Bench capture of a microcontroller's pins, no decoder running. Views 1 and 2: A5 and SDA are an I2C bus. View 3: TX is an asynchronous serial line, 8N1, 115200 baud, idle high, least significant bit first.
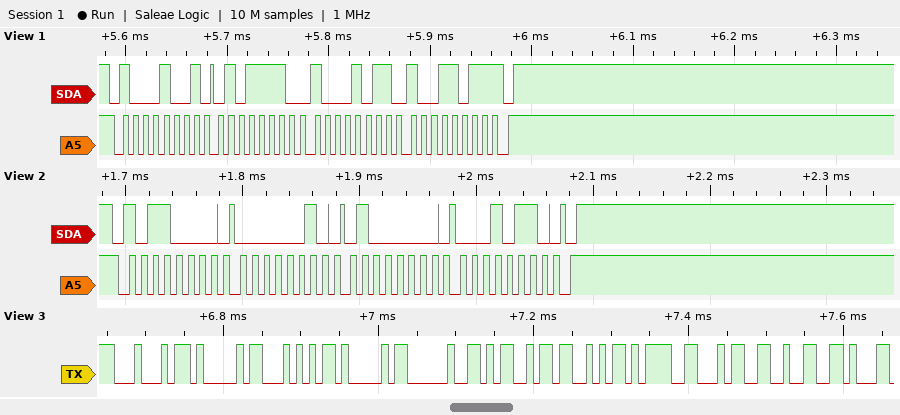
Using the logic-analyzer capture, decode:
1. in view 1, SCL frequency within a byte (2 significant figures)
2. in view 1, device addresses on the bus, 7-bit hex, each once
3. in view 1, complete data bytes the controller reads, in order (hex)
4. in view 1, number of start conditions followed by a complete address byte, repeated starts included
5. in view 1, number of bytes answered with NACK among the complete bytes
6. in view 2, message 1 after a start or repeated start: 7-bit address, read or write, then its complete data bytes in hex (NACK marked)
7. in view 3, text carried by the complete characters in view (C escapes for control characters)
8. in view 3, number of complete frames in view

100 kHz
0x44
5E 8B 9B
1
1
0x58 write: 02 40 16
"DATA MS=42"
10
